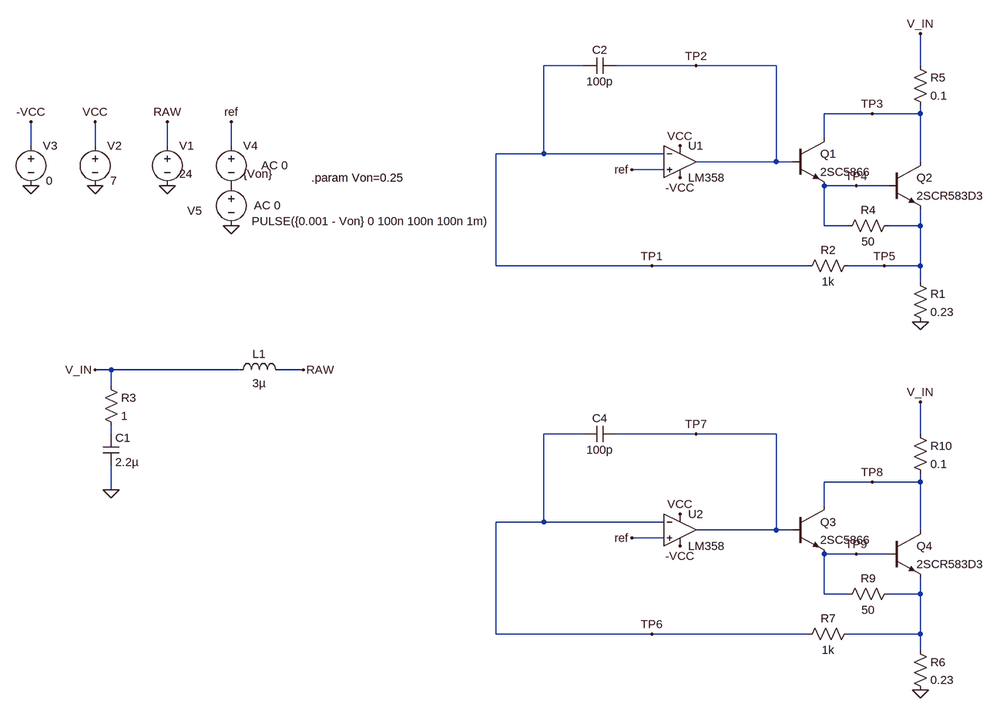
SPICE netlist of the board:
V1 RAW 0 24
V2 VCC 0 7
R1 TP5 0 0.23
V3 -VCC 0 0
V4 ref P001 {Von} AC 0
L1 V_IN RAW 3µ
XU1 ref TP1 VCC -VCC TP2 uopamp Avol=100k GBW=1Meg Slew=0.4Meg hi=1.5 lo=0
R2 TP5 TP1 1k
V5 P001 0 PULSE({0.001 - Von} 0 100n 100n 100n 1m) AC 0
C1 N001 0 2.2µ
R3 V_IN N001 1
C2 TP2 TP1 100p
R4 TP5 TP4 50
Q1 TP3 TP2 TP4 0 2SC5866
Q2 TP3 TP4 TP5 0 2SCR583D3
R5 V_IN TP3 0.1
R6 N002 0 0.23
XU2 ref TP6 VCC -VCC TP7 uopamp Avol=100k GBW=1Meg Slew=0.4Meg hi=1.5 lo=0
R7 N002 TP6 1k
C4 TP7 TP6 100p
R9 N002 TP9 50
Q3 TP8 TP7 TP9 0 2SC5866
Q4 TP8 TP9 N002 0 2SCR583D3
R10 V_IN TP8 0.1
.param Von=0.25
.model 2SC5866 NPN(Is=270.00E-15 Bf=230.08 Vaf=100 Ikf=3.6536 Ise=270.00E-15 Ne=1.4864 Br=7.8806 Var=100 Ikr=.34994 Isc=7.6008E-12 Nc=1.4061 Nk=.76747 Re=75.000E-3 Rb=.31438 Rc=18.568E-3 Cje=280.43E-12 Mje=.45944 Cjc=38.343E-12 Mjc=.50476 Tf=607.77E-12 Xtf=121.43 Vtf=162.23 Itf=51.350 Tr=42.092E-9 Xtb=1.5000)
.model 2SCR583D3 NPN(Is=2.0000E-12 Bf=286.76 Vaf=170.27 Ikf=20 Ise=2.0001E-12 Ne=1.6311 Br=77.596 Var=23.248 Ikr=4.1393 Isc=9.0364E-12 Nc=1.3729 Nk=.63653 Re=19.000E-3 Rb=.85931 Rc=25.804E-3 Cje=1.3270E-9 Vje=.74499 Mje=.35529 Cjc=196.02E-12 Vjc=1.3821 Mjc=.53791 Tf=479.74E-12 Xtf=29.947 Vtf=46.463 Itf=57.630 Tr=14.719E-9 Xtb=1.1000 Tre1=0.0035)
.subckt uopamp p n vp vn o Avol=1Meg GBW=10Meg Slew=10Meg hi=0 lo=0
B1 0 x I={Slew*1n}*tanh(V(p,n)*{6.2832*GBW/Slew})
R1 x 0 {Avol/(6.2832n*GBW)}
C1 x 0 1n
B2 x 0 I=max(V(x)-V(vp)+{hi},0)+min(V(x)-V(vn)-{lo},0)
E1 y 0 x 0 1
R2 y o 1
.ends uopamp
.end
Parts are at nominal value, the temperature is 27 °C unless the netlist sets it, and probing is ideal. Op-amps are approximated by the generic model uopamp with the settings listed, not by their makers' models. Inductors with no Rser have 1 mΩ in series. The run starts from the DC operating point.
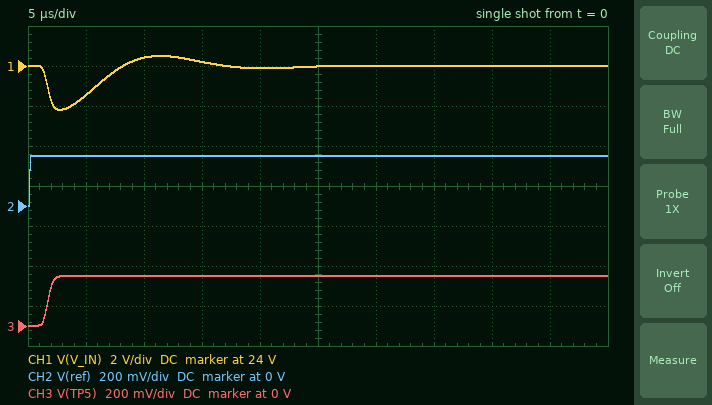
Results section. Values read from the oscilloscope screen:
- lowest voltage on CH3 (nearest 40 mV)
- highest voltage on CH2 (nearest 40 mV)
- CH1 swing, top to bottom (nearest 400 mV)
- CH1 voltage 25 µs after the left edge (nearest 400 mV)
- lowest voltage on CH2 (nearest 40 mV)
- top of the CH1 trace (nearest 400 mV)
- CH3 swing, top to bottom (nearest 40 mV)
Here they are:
0 V
240 mV
2.8 V
24.0 V
0 V
24.4 V
240 mV
